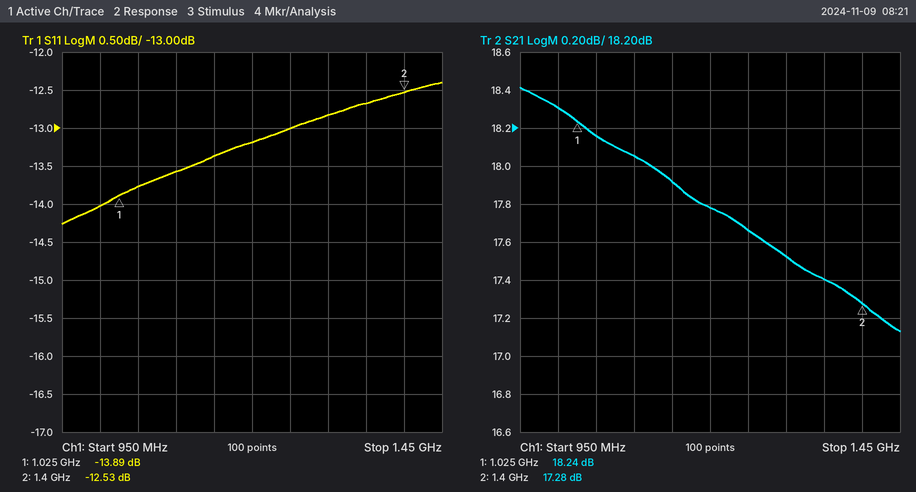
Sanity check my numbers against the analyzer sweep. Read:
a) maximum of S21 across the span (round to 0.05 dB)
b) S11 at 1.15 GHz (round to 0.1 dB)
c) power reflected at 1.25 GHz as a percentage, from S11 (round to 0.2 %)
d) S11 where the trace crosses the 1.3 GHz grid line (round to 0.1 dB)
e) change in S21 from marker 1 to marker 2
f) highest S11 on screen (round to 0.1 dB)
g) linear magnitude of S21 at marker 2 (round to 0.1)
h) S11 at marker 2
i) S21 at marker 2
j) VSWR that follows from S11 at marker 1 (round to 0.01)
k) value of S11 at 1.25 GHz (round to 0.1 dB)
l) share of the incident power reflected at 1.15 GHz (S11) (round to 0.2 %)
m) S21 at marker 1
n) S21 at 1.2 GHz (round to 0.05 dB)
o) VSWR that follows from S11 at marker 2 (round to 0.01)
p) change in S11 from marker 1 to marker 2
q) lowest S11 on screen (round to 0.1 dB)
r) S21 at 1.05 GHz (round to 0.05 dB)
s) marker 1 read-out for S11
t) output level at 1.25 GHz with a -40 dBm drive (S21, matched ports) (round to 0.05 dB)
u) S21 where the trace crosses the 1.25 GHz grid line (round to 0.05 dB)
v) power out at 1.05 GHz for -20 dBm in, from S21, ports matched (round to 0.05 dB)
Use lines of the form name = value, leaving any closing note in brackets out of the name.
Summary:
maximum of S21 across the span = 18.40 dB
S11 at 1.15 GHz = -13.4 dB
power reflected at 1.25 GHz as a percentage, from S11 = 5.0 %
S11 where the trace crosses the 1.3 GHz grid line = -12.8 dB
change in S21 from marker 1 to marker 2 = -0.96 dB
highest S11 on screen = -12.4 dB
linear magnitude of S21 at marker 2 = 7.3
S11 at marker 2 = -12.53 dB
S21 at marker 2 = 17.28 dB
VSWR that follows from S11 at marker 1 = 1.51
value of S11 at 1.25 GHz = -13.0 dB
share of the incident power reflected at 1.15 GHz (S11) = 4.6 %
S21 at marker 1 = 18.24 dB
S21 at 1.2 GHz = 17.80 dB
VSWR that follows from S11 at marker 2 = 1.62
change in S11 from marker 1 to marker 2 = 1.36 dB
lowest S11 on screen = -14.3 dB
S21 at 1.05 GHz = 18.15 dB
marker 1 read-out for S11 = -13.89 dB
output level at 1.25 GHz with a -40 dBm drive (S21, matched ports) = -22.35 dBm
S21 where the trace crosses the 1.25 GHz grid line = 17.65 dB
power out at 1.05 GHz for -20 dBm in, from S21, ports matched = -1.85 dBm
